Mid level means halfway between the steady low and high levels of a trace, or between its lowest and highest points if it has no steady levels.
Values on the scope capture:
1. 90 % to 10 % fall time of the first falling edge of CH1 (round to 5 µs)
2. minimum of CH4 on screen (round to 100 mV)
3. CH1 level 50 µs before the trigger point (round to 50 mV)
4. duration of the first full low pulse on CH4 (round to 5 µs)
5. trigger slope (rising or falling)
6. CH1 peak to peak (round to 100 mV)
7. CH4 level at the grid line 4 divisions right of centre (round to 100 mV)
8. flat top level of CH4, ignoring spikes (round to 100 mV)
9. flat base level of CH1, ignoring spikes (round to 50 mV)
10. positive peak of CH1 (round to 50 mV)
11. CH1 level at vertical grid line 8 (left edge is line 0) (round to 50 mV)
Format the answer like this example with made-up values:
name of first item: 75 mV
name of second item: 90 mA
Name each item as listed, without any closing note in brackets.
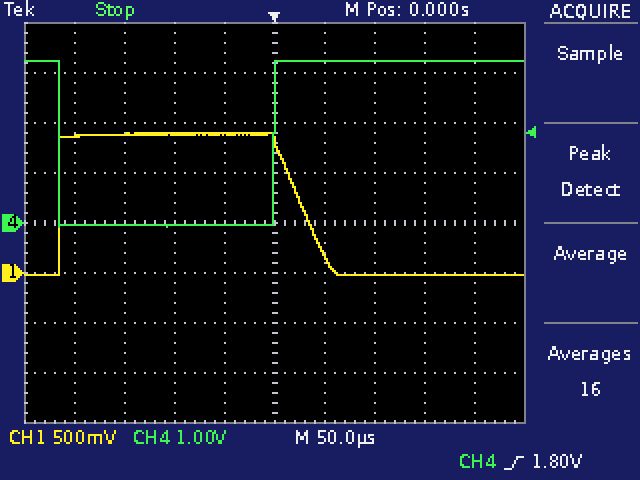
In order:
90 % to 10 % fall time of the first falling edge of CH1: 50 µs
minimum of CH4 on screen: -100 mV
CH1 level 50 µs before the trigger point: 1.40 V
duration of the first full low pulse on CH4: 215 µs
trigger slope: rising
CH1 peak to peak: 1.40 V
CH4 level at the grid line 4 divisions right of centre: 3.2 V
flat top level of CH4, ignoring spikes: 3.2 V
flat base level of CH1, ignoring spikes: 0 mV
positive peak of CH1: 1.40 V
CH1 level at vertical grid line 8 (left edge is line 0): 0 mV
